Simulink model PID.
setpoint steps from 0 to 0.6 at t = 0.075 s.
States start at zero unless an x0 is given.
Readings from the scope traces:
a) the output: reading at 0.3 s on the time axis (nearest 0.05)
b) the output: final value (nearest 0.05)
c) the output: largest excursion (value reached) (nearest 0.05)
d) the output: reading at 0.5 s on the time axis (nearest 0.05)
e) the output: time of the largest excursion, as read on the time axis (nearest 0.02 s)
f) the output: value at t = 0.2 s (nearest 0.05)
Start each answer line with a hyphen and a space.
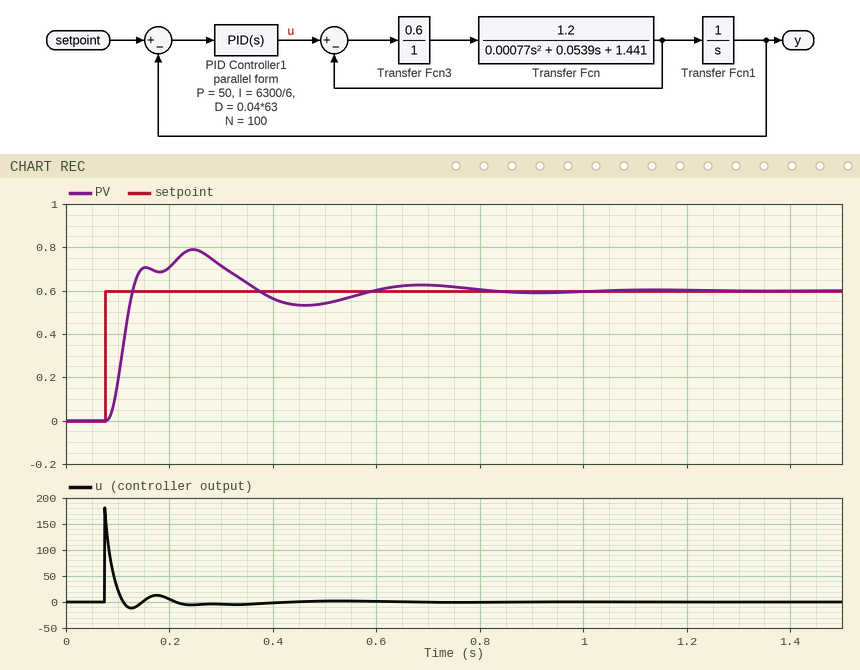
- 0.70
- 0.60
- 0.80
- 0.55
- 0.24 s
- 0.70
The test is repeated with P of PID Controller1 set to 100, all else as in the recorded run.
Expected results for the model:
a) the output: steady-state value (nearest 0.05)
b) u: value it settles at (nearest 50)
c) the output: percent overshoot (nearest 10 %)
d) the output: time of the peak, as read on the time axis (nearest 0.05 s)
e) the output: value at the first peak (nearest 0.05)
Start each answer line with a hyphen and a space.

- 0.60
- 0
- 40 %
- 0.15 s
- 0.85
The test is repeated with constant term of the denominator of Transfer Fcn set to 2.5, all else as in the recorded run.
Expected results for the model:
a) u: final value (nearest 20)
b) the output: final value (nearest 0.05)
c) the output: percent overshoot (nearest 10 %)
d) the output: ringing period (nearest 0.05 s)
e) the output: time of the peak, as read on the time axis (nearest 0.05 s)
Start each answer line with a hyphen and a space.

- 0
- 0.60
- 30 %
- 0.50 s
- 0.30 s
